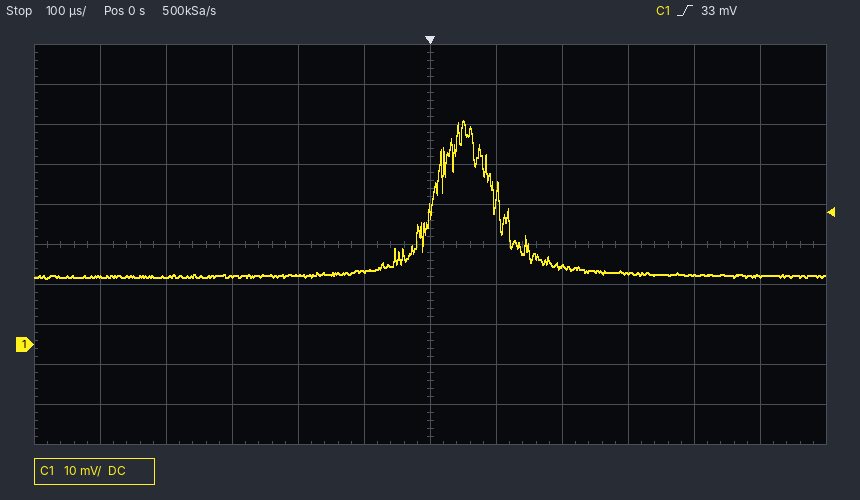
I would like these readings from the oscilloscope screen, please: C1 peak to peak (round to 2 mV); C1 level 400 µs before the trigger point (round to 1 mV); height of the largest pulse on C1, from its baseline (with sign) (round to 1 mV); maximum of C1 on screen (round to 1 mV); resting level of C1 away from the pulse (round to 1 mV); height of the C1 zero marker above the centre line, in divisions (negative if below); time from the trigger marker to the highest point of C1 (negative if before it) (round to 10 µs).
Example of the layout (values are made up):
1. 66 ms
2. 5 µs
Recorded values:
1. 40 mV
2. 17 mV
3. +39 mV
4. 56 mV
5. 17 mV
6. -2.5 div
7. +50 µs
